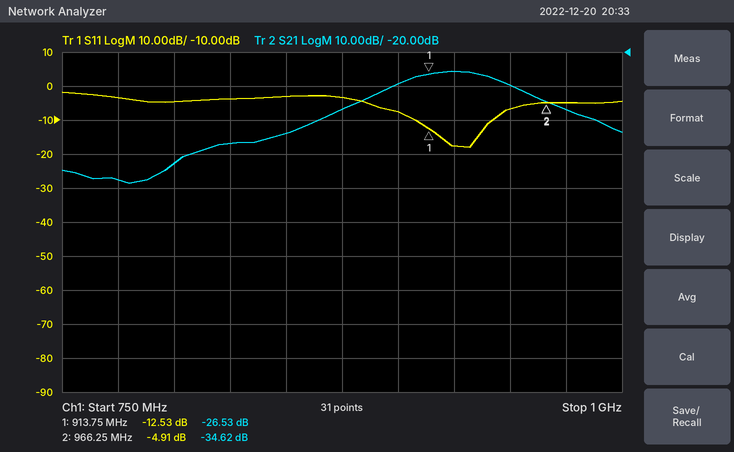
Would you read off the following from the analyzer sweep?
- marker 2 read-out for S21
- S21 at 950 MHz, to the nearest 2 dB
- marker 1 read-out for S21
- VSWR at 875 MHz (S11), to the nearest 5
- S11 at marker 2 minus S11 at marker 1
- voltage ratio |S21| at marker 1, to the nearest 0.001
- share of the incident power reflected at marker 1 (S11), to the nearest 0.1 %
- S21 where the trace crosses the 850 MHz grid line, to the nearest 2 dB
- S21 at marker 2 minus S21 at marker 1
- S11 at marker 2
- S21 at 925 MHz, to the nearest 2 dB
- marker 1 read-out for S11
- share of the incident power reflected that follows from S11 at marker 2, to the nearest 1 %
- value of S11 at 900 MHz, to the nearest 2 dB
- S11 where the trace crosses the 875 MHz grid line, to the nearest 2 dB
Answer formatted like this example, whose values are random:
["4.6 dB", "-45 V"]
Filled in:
["-34.62 dB", "-30 dB", "-26.53 dB", "5", "7.62 dB", "0.047", "5.6 %", "-44 dB", "-8.09 dB", "-4.91 dB", "-26 dB", "-12.53 dB", "32 %", "-8 dB", "-4 dB"]
